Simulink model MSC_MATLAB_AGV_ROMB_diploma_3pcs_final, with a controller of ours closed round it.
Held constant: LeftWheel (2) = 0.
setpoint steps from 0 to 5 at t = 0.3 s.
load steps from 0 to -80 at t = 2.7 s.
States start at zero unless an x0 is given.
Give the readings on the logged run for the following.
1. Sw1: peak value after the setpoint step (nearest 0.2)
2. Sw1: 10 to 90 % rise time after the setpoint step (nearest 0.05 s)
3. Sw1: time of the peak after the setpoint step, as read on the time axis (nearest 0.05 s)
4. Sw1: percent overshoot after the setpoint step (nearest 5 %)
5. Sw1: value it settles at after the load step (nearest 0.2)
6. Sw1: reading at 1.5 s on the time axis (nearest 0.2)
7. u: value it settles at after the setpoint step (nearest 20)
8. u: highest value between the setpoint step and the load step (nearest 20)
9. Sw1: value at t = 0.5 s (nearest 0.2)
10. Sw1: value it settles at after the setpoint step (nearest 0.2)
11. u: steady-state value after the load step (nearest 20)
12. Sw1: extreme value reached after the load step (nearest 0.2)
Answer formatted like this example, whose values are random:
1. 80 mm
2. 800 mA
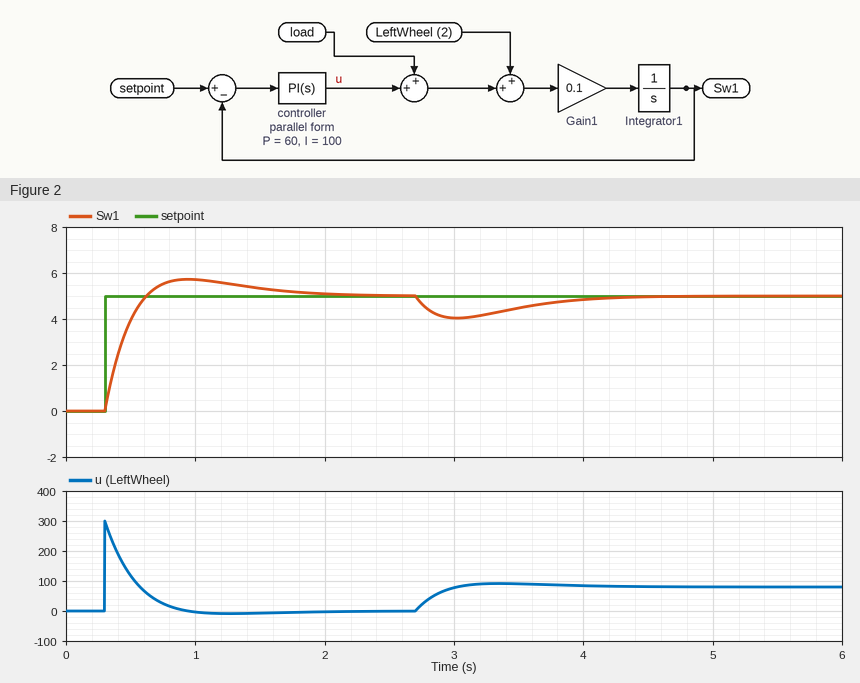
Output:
1. 5.8
2. 0.25 s
3. 0.95 s
4. 15 %
5. 5.0
6. 5.4
7. 0
8. 300
9. 4.0
10. 5.0
11. 80
12. 4.0
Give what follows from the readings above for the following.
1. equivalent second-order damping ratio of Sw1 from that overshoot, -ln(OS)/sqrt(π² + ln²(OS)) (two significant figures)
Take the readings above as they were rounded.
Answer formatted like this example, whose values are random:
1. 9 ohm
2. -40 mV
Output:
1. 0.52
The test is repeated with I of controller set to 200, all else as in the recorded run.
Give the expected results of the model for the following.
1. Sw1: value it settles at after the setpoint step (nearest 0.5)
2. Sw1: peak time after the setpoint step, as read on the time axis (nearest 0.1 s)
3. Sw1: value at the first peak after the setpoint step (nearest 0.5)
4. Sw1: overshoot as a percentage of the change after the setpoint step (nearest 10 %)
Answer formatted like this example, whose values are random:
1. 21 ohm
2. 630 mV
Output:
1. 5.0
2. 0.8 s
3. 6.0
4. 20 %
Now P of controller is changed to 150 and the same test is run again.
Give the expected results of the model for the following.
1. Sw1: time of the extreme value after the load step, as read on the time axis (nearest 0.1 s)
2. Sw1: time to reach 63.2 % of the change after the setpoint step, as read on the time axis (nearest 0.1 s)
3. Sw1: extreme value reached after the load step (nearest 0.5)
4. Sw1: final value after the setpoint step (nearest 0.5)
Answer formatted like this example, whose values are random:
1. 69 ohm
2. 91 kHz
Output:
1. 2.9 s
2. 0.4 s
3. 4.5
4. 5.0
